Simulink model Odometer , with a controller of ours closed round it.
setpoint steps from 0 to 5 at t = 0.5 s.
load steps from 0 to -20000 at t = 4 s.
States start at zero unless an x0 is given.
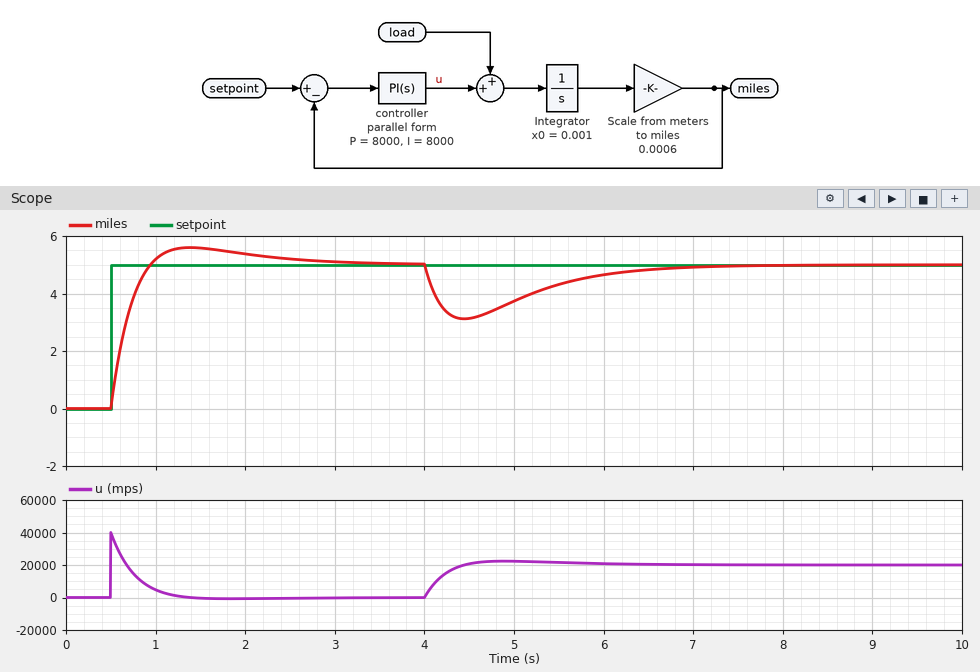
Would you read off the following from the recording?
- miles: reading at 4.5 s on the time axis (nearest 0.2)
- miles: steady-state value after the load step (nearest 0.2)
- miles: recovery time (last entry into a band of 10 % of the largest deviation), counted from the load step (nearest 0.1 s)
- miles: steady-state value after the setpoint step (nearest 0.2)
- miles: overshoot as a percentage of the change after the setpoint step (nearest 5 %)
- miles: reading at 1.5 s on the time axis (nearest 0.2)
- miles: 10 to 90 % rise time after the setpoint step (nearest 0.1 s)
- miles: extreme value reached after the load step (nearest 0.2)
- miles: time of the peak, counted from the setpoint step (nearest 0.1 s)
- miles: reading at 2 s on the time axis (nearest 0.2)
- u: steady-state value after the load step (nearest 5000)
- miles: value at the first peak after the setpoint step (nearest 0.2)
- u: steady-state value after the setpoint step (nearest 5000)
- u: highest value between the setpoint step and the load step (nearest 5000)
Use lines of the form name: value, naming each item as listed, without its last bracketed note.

miles: reading at 4.5 s on the time axis: 3.2
miles: steady-state value after the load step: 5.0
miles: recovery time (last entry into a band of 10 % of the largest deviation), counted from the load step: 2.4 s
miles: steady-state value after the setpoint step: 5.0
miles: overshoot as a percentage of the change after the setpoint step: 10 %
miles: reading at 1.5 s on the time axis: 5.6
miles: 10 to 90 % rise time after the setpoint step: 0.3 s
miles: extreme value reached after the load step: 3.2
miles: time of the peak, counted from the setpoint step: 0.9 s
miles: reading at 2 s on the time axis: 5.4
u: steady-state value after the load step: 20000
miles: value at the first peak after the setpoint step: 5.6
u: steady-state value after the setpoint step: 0
u: highest value between the setpoint step and the load step: 40000
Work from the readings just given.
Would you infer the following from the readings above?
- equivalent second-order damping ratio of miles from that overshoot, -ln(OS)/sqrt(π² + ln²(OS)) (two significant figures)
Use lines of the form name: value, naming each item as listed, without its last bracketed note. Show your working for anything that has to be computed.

equivalent second-order damping ratio of miles from that overshoot, -ln(OS)/sqrt(π² + ln²(OS)): ln(0.1) = -2.303; 2.303 / sqrt(9.870 + 5.302) = 0.59
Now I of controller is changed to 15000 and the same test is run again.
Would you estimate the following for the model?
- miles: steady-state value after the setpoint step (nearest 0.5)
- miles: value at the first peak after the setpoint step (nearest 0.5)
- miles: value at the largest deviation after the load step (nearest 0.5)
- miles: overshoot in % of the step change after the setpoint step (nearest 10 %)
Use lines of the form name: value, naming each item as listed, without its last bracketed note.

miles: steady-state value after the setpoint step: 5.0
miles: value at the first peak after the setpoint step: 6.0
miles: value at the largest deviation after the load step: 3.5
miles: overshoot in % of the step change after the setpoint step: 20 %
